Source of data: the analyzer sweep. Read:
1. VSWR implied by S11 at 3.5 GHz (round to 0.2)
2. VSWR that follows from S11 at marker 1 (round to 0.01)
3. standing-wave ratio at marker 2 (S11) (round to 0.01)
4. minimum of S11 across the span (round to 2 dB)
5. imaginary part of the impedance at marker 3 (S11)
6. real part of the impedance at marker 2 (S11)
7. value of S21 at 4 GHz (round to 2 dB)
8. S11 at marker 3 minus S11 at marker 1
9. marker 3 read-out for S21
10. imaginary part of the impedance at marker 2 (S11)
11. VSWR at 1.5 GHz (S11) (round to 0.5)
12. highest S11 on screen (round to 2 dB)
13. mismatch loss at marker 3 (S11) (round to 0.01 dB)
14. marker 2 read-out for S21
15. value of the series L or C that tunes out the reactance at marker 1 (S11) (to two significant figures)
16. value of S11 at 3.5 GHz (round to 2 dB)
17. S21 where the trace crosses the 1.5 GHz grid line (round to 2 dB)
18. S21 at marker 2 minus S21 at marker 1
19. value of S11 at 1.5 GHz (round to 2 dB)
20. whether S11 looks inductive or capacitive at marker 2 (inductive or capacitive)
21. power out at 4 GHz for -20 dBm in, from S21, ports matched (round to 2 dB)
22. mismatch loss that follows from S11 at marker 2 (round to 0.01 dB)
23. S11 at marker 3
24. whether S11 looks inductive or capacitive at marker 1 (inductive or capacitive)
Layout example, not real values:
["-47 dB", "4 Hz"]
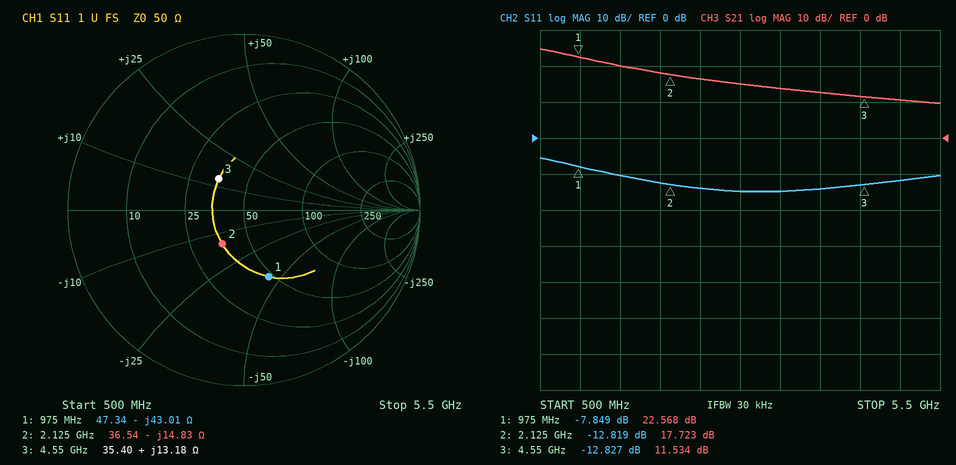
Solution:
["1.4", "2.36", "1.59", "-14 dB", "+13.18 Ω", "36.54 Ω", "12 dB", "-4.978 dB", "11.534 dB", "-14.83 Ω", "2.0", "-6 dB", "0.23 dB", "17.723 dB", "7.0 nH", "-14 dB", "20 dB", "-4.845 dB", "-10 dB", "capacitive", "-8 dBm", "0.23 dB", "-12.827 dB", "capacitive"]
